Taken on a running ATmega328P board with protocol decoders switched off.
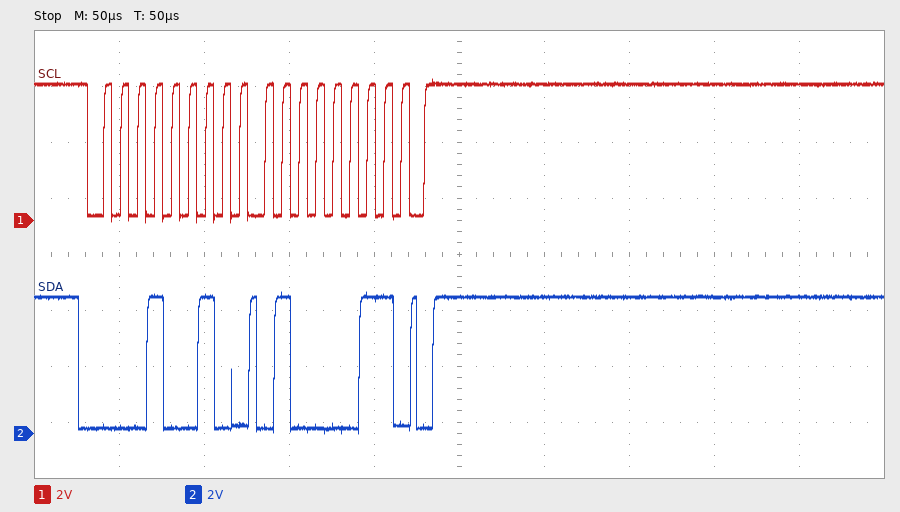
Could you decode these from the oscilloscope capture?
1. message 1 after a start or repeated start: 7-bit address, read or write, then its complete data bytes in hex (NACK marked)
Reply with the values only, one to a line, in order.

0x09 write: 43
